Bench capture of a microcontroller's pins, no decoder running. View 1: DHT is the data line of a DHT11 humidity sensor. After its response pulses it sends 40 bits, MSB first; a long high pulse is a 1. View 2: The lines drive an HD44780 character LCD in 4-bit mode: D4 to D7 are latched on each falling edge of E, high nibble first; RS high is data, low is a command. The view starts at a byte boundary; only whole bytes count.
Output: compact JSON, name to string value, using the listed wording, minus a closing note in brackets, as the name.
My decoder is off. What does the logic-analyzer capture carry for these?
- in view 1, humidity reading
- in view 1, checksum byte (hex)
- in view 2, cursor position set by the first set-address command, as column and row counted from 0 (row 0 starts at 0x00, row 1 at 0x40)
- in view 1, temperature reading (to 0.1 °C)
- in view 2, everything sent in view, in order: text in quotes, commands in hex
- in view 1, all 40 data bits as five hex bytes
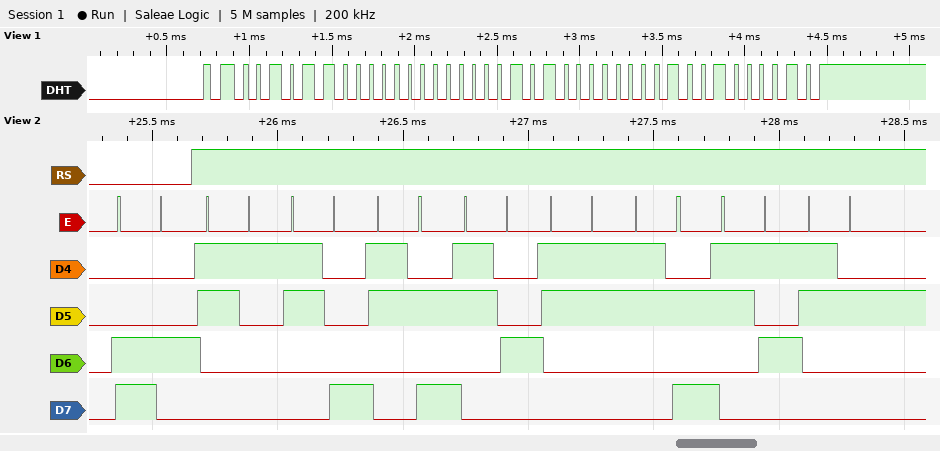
{"in view 1, humidity reading": "44 %", "in view 1, checksum byte": "0x42", "in view 2, cursor position set by the first set-address command, as column and row counted from 0": "column 4, row 1", "in view 1, temperature reading": "20.2 °C", "in view 2, everything sent in view, in order: text in quotes, commands in hex": "0xC4 \"18:43:52\"", "in view 1, all 40 data bits as five hex bytes": "2C 00 14 02 42"}
